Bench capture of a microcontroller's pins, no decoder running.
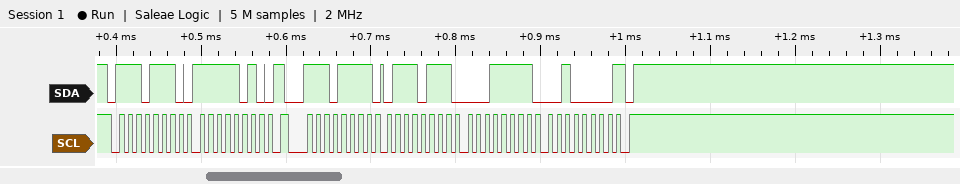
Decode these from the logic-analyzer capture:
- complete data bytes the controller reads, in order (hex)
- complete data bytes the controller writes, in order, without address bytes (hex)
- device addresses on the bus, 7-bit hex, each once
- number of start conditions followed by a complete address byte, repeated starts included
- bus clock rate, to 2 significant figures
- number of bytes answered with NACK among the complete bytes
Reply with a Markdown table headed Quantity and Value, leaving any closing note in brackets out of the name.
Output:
| Quantity | Value |
|---|---|
| complete data bytes the controller reads, in order | 77 1F 20 |
| complete data bytes the controller writes, in order, without address bytes | FA |
| device addresses on the bus, 7-bit hex, each once | 0x77 |
| number of start conditions followed by a complete address byte, repeated starts included | 2 |
| bus clock rate, to 2 significant figures | 100 kHz |
| number of bytes answered with NACK among the complete bytes | 1 |
